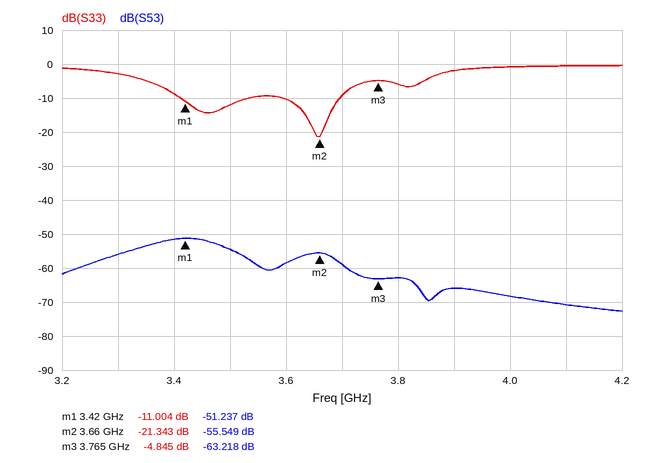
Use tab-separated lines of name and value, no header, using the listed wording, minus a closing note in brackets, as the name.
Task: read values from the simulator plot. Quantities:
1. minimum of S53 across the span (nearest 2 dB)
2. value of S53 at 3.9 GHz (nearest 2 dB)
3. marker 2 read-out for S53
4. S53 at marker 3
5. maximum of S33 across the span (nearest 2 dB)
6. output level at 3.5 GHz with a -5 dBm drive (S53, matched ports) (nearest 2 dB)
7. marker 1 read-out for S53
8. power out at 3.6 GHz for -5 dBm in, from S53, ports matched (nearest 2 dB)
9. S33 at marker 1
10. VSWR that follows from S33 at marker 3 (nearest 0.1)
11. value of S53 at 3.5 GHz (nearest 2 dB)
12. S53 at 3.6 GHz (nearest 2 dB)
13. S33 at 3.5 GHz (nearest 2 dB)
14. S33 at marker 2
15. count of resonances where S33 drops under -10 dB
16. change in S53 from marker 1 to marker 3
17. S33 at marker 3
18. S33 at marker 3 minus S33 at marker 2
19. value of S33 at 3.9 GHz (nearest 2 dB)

minimum of S53 across the span	-72 dB
value of S53 at 3.9 GHz	-66 dB
marker 2 read-out for S53	-55.549 dB
S53 at marker 3	-63.218 dB
maximum of S33 across the span	0 dB
output level at 3.5 GHz with a -5 dBm drive (S53, matched ports)	-60 dBm
marker 1 read-out for S53	-51.237 dB
power out at 3.6 GHz for -5 dBm in, from S53, ports matched	-64 dBm
S33 at marker 1	-11.004 dB
VSWR that follows from S33 at marker 3	3.7
value of S53 at 3.5 GHz	-54 dB
S53 at 3.6 GHz	-58 dB
S33 at 3.5 GHz	-12 dB
S33 at marker 2	-21.343 dB
count of resonances where S33 drops under -10 dB	2
change in S53 from marker 1 to marker 3	-11.981 dB
S33 at marker 3	-4.845 dB
S33 at marker 3 minus S33 at marker 2	16.498 dB
value of S33 at 3.9 GHz	-2 dB
